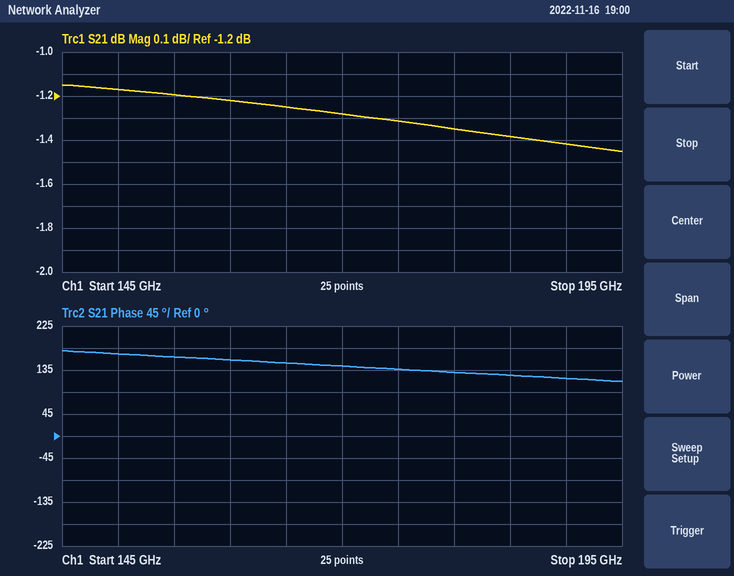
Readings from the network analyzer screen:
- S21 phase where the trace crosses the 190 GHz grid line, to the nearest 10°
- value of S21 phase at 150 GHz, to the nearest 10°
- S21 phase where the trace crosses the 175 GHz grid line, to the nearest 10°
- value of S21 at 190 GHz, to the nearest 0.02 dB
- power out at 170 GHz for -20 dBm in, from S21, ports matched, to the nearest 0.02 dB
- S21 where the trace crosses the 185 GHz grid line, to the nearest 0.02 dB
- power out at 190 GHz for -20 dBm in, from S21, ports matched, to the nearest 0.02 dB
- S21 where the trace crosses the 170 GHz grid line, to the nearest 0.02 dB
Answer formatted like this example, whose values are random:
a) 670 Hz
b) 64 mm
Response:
a) 120°
b) 170°
c) 140°
d) -1.42 dB
e) -21.28 dBm
f) -1.38 dB
g) -21.42 dBm
h) -1.28 dB
